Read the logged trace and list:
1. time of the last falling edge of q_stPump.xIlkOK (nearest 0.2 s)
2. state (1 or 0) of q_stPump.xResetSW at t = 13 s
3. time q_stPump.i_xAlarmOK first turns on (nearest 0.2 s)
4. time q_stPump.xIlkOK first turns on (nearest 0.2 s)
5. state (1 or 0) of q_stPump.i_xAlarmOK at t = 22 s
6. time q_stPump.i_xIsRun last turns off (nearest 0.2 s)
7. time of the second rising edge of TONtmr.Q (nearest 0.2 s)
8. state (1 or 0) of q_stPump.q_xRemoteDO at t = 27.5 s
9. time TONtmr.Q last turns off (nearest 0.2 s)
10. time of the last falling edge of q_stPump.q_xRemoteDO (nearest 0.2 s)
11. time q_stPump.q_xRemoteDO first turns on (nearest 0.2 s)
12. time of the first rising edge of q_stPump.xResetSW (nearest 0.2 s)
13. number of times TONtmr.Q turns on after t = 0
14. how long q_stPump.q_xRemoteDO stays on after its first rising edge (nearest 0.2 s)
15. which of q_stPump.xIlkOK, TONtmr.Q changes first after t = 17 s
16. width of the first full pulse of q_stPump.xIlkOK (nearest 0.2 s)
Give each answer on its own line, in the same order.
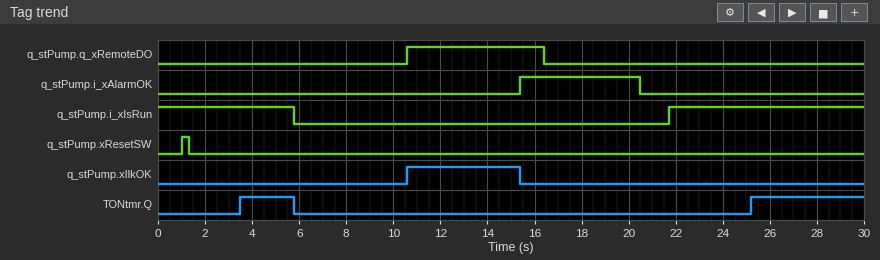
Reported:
15.4 s
0
15.4 s
10.6 s
0
5.8 s
25.2 s
0
5.8 s
16.4 s
10.6 s
1.0 s
2
5.8 s
TONtmr.Q
4.8 s
